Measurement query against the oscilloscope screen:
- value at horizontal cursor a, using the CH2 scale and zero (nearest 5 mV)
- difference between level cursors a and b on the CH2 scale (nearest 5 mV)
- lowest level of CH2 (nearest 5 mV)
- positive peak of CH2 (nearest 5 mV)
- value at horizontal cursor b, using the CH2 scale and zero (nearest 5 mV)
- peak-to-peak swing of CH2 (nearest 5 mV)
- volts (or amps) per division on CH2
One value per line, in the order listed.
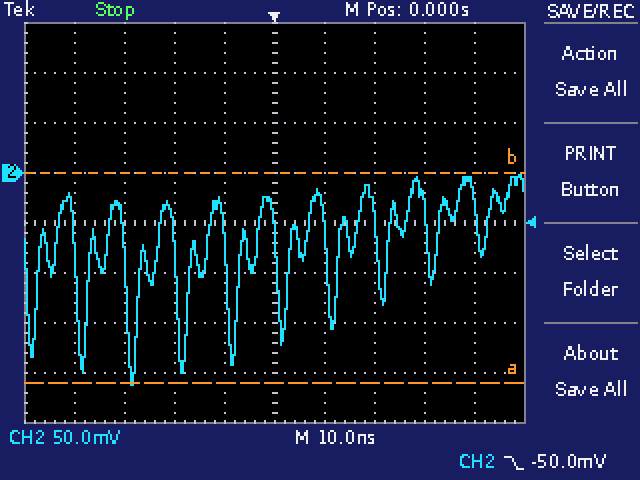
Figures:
-210 mV
210 mV
-210 mV
0 mV
0 mV
210 mV
50 mV
